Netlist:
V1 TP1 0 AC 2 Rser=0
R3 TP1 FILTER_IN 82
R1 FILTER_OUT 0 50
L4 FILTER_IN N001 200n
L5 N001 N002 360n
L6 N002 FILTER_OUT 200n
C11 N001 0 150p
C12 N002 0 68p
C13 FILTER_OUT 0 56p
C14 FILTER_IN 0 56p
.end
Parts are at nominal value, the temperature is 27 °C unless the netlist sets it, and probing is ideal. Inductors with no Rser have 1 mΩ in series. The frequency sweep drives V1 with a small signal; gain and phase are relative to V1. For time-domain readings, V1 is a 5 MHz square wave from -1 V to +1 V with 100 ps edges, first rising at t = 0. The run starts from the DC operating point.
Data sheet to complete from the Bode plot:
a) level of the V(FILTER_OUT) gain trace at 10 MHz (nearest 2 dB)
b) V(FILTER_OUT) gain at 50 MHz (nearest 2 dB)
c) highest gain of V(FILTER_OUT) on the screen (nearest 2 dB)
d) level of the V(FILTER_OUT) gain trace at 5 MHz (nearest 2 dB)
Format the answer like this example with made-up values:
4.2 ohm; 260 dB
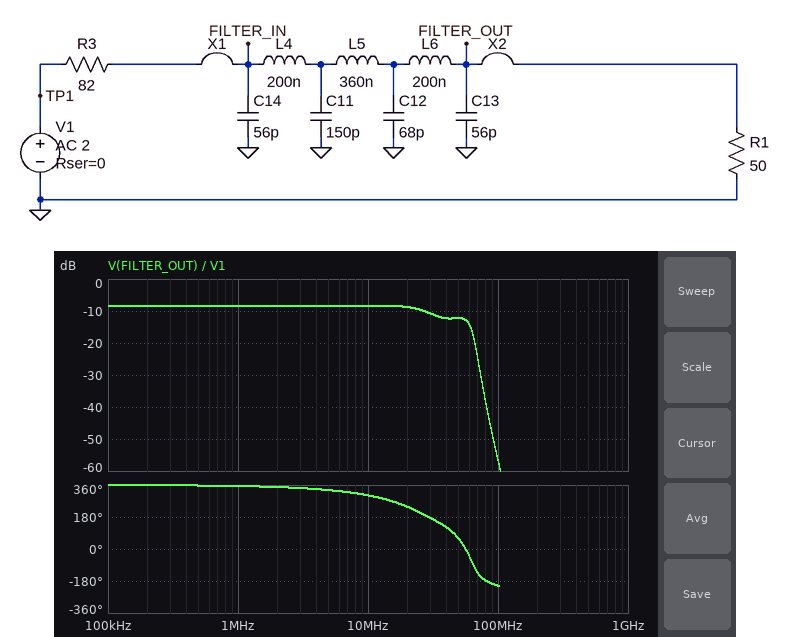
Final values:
-8 dB; -12 dB; -8 dB; -8 dB
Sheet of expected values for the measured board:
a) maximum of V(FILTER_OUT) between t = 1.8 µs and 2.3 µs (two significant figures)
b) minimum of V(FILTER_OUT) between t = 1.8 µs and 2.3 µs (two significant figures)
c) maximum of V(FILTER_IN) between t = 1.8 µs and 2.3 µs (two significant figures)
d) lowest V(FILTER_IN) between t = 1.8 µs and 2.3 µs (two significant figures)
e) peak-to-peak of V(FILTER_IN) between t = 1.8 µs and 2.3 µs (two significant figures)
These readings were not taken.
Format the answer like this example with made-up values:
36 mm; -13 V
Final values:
430 mV; -430 mV; 640 mV; -640 mV; 1.3 V
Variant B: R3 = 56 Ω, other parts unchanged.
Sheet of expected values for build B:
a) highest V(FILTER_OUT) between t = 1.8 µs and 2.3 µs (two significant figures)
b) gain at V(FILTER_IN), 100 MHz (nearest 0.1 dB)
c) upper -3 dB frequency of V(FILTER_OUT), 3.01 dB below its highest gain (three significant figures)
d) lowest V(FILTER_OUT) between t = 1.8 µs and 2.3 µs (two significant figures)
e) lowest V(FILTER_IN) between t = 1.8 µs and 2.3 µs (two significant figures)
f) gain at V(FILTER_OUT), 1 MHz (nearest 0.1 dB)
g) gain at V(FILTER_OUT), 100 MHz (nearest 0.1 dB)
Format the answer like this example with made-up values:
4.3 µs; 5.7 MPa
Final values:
550 mV; -5.0 dB; 39.3 MHz; -550 mV; -730 mV; -6.5 dB; -54.1 dB
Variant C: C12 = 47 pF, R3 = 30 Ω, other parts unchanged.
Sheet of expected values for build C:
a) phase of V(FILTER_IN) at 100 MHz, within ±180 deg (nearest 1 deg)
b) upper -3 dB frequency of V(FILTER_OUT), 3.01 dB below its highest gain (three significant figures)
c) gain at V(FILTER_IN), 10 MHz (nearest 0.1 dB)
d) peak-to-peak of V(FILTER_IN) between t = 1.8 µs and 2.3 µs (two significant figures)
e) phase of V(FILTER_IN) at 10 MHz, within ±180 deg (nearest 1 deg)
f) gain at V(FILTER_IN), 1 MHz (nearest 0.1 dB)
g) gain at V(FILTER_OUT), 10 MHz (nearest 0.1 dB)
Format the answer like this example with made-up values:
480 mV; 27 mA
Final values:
-38 deg; 40.6 MHz; -3.7 dB; 1.8 V; -2 deg; -4.1 dB; -4.2 dB
